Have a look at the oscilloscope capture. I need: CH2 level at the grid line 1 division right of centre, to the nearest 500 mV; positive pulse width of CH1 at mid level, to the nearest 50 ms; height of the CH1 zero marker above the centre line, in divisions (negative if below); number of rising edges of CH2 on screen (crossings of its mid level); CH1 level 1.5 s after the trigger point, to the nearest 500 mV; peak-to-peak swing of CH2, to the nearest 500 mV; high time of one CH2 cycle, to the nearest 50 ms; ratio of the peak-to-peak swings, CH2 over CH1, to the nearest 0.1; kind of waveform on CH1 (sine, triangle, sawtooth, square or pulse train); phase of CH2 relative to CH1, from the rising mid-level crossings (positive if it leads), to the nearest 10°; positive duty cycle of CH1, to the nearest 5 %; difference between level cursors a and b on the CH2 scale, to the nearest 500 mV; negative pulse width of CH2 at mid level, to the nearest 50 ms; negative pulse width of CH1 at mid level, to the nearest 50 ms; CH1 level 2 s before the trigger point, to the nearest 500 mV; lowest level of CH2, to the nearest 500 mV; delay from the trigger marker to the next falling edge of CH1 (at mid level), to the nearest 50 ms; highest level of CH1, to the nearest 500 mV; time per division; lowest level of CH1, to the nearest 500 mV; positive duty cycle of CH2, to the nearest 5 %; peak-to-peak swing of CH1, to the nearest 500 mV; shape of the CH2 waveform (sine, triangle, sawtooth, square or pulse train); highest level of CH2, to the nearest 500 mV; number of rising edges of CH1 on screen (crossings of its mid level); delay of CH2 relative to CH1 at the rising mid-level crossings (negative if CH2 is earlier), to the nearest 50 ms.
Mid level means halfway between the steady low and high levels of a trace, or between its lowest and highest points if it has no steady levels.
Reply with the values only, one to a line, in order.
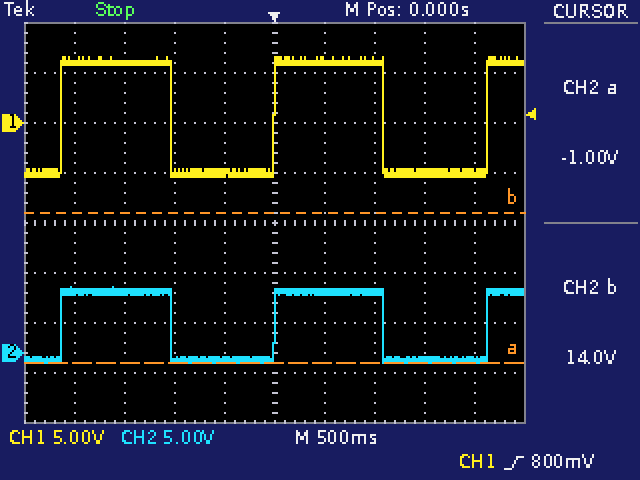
6.0 V
1.10 s
+2.0 div
3
-5.0 V
7.5 V
1.10 s
0.6
square
0°
50 %
15.0 V
1.05 s
1.05 s
6.0 V
-1.0 V
1.10 s
6.5 V
500 ms
-5.5 V
50 %
12.0 V
square
6.5 V
3
0 ms
